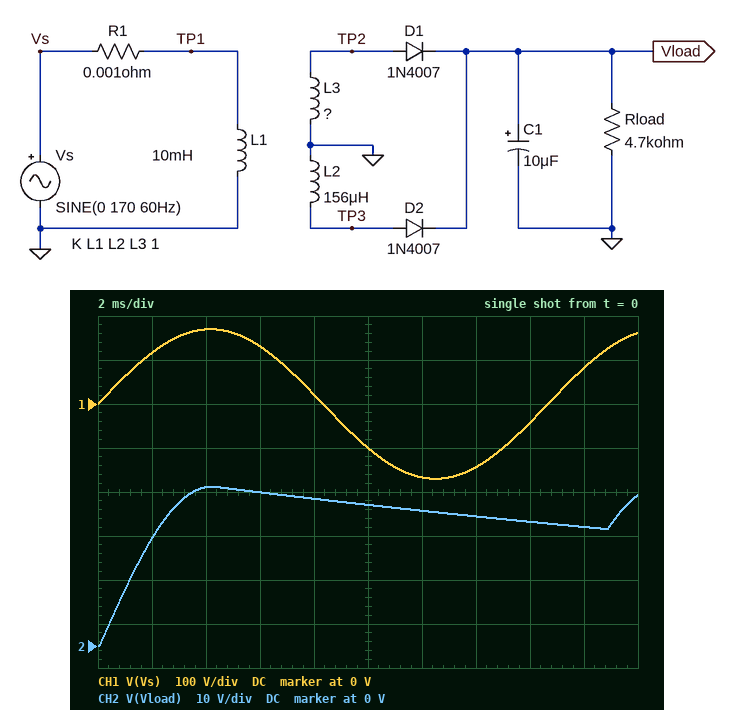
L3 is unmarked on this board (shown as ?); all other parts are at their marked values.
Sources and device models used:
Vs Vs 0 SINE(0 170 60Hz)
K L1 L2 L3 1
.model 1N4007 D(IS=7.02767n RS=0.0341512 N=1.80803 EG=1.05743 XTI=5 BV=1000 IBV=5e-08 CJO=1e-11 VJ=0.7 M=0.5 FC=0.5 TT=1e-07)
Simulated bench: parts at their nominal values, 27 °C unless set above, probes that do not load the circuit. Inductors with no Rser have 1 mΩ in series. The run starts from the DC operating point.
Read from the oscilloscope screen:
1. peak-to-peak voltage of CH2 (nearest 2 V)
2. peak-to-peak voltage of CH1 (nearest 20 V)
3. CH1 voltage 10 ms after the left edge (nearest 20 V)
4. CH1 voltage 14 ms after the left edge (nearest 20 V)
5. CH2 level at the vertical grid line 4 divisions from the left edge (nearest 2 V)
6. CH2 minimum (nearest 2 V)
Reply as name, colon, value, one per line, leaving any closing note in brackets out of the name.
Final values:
peak-to-peak voltage of CH2: 36 V
peak-to-peak voltage of CH1: 340 V
CH1 voltage 10 ms after the left edge: -100 V
CH1 voltage 14 ms after the left edge: -140 V
CH2 level at the vertical grid line 4 divisions from the left edge: 34 V
CH2 minimum: 0 V
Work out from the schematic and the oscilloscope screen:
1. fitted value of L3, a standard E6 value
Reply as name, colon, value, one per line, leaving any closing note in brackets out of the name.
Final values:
fitted value of L3, a standard E6 value: 470 µH
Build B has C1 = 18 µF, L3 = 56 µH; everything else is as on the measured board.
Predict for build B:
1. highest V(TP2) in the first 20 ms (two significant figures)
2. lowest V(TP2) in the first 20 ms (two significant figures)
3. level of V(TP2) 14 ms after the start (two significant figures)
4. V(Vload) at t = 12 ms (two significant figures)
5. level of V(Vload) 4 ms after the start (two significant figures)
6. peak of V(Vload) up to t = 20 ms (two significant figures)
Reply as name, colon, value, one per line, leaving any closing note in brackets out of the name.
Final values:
highest V(TP2) in the first 20 ms: 13 V
lowest V(TP2) in the first 20 ms: -13 V
level of V(TP2) 14 ms after the start: -11 V
V(Vload) at t = 12 ms: 20 V
level of V(Vload) 4 ms after the start: 12 V
peak of V(Vload) up to t = 20 ms: 21 V
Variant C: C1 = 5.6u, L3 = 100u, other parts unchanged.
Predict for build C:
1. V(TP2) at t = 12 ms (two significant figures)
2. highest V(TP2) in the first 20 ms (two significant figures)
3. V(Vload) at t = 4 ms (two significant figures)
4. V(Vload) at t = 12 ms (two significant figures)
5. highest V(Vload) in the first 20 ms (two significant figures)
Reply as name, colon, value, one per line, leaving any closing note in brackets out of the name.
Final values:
V(TP2) at t = 12 ms: -17 V
highest V(TP2) in the first 20 ms: 17 V
V(Vload) at t = 4 ms: 16 V
V(Vload) at t = 12 ms: 20 V
highest V(Vload) in the first 20 ms: 21 V
